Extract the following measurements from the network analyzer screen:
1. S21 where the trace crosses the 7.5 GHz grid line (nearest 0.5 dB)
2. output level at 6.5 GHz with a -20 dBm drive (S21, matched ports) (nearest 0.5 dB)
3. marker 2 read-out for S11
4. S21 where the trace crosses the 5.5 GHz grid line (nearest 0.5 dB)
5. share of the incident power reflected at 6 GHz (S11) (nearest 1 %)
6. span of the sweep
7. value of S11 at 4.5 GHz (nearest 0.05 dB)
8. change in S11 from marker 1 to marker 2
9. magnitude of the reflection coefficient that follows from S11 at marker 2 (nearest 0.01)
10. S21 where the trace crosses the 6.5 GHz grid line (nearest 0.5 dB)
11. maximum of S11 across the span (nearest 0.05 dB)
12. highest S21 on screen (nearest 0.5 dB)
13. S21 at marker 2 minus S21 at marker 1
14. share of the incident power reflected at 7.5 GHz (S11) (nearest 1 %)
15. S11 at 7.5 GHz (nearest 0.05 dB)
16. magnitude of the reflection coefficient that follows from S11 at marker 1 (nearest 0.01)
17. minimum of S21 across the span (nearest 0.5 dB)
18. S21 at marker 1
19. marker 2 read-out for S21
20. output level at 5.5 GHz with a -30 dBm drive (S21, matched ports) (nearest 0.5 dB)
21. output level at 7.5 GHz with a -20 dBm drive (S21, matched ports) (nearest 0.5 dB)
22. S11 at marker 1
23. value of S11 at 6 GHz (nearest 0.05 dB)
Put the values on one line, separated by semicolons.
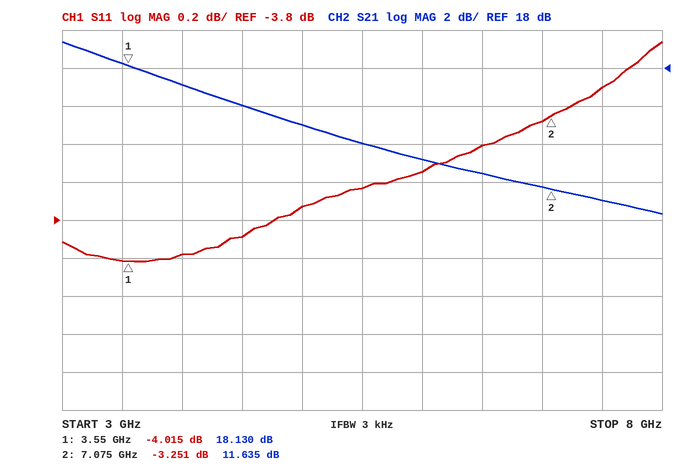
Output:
11.0 dB; -7.5 dBm; -3.251 dB; 14.0 dB; 44 %; 5 GHz; -3.90 dB; 0.764 dB; 0.69; 12.5 dB; -2.85 dB; 19.5 dB; -6.495 dB; 49 %; -3.10 dB; 0.63; 10.5 dB; 18.130 dB; 11.635 dB; -16.0 dBm; -9.0 dBm; -4.015 dB; -3.55 dB
